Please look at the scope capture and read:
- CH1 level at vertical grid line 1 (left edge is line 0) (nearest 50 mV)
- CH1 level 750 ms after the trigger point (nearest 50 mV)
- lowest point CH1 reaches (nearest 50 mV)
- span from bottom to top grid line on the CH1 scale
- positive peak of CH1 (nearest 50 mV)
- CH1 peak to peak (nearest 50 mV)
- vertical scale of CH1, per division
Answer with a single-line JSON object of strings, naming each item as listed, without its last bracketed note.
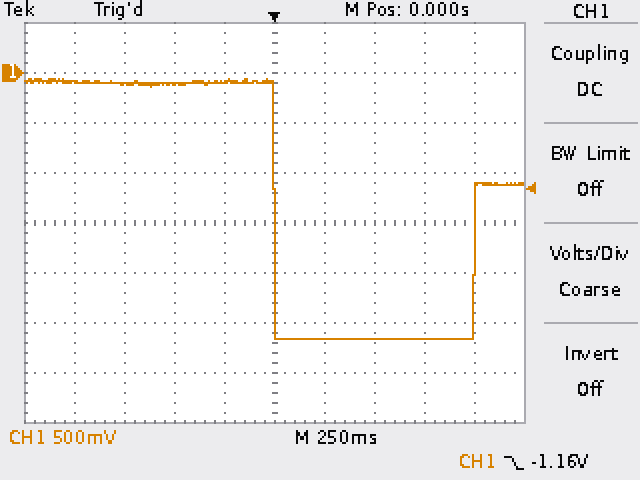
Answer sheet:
{"CH1 level at vertical grid line 1 (left edge is line 0)": "-100 mV", "CH1 level 750 ms after the trigger point": "-2.65 V", "lowest point CH1 reaches": "-2.65 V", "span from bottom to top grid line on the CH1 scale": "4 V", "positive peak of CH1": "-50 mV", "CH1 peak to peak": "2.60 V", "vertical scale of CH1, per division": "500 mV"}
